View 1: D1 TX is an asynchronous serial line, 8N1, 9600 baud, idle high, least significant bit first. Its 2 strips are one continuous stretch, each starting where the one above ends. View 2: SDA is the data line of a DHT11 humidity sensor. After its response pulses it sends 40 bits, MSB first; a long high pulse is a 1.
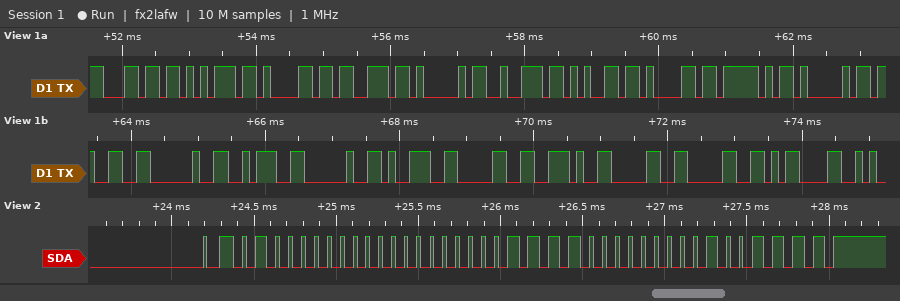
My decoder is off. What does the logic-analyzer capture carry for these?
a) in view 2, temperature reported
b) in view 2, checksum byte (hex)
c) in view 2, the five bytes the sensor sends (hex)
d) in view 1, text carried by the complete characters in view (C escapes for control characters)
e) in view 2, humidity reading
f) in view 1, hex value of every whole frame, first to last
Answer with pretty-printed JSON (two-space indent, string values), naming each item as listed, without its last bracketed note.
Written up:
{
  "in view 2, temperature reported": "15.0 °C",
  "in view 2, checksum byte": "0x4F",
  "in view 2, the five bytes the sensor sends": "40 00 0F 00 4F",
  "in view 1, text carried by the complete characters in view": "\"luasArea_A3 : 90.00\\r\"",
  "in view 2, humidity reading": "64 %",
  "in view 1, hex value of every whole frame, first to last": "0x6C 0x75 0x61 0x73 0x41 0x72 0x65 0x61 0x5F 0x41 0x33 0x20 0x3A 0x20 0x39 0x30 0x2E 0x30 0x30 0x0D"
}
